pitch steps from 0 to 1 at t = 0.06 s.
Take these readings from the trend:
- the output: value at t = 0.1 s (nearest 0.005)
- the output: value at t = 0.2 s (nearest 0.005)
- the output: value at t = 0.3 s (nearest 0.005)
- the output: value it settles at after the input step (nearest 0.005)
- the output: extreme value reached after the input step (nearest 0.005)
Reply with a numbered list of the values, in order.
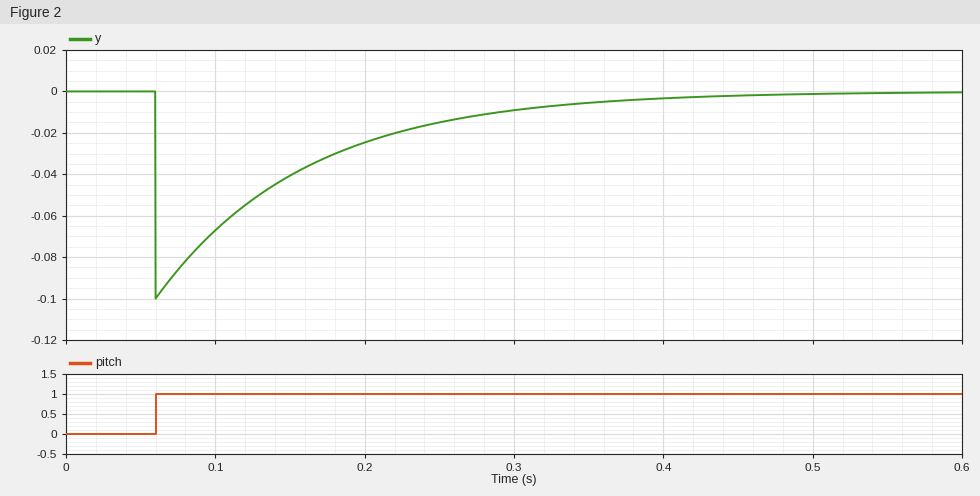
1. -0.065
2. -0.025
3. -0.010
4. 0.000
5. -0.100
